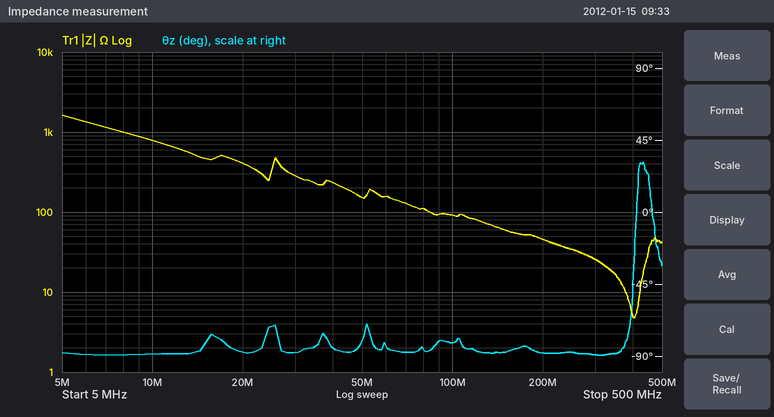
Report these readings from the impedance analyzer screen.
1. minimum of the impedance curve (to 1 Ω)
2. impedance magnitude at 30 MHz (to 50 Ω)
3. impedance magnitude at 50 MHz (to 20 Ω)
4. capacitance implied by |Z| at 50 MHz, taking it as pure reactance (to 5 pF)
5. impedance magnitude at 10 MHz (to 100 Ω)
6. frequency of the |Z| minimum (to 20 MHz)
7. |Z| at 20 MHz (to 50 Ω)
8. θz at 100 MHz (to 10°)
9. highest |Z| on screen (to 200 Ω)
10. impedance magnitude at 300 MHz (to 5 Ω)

5 Ω
300 Ω
160 Ω
20 pF
800 Ω
400 MHz
400 Ω
-80°
1.6 kΩ
25 Ω
